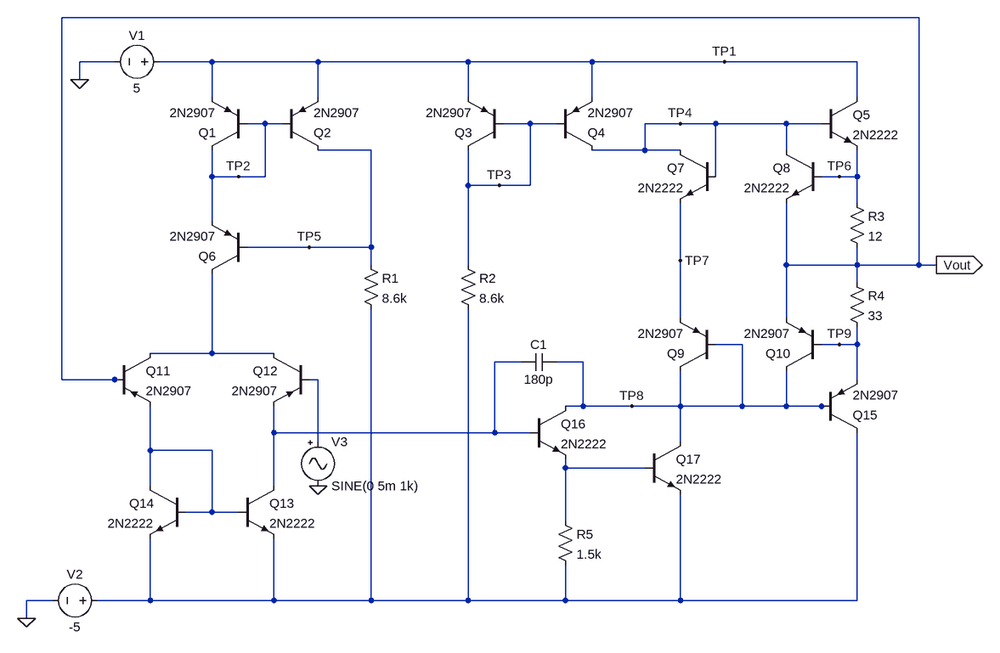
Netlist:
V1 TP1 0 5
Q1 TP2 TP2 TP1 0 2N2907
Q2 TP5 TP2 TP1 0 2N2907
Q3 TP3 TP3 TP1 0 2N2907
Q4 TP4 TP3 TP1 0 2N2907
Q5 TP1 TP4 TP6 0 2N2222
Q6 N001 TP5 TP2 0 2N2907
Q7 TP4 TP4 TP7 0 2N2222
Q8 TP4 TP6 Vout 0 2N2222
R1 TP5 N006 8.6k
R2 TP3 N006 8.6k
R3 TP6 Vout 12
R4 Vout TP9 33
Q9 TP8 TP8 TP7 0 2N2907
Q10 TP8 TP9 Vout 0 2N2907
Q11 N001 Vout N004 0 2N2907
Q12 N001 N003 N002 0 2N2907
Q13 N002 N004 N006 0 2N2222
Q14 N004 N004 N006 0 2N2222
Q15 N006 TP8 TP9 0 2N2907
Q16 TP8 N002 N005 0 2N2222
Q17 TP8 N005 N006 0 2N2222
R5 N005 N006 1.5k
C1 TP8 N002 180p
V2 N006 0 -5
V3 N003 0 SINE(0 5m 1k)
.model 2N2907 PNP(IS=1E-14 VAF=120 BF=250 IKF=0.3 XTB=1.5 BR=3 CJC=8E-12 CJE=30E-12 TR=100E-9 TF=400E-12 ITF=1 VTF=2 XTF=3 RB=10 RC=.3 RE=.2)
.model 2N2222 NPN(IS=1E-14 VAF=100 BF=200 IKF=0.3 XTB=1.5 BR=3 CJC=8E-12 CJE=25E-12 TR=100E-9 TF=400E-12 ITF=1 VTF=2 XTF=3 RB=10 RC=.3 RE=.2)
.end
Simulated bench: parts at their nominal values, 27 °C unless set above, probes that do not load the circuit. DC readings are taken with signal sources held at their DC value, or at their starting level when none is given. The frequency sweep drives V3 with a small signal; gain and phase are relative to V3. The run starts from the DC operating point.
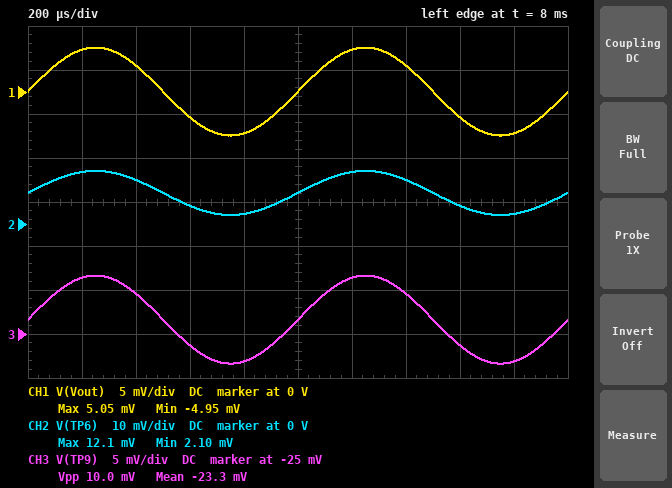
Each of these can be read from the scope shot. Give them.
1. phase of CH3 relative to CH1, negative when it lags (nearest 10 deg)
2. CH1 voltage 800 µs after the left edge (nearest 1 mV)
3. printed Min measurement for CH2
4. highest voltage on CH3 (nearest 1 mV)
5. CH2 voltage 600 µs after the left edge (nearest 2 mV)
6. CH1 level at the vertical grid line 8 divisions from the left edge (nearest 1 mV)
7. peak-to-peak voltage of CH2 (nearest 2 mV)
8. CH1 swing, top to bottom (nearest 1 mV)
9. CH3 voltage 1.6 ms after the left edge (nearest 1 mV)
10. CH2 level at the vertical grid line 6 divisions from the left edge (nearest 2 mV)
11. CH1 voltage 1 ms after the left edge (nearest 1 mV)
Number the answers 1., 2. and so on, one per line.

1. 0 deg
2. -5 mV
3. 2.10 mV
4. -18 mV
5. 4 mV
6. -3 mV
7. 10 mV
8. 10 mV
9. -26 mV
10. 12 mV
11. 0 V
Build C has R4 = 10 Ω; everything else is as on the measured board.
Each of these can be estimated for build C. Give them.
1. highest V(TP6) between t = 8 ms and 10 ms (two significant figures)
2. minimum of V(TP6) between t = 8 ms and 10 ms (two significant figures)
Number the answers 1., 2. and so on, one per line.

1. 14 mV
2. 4.1 mV
